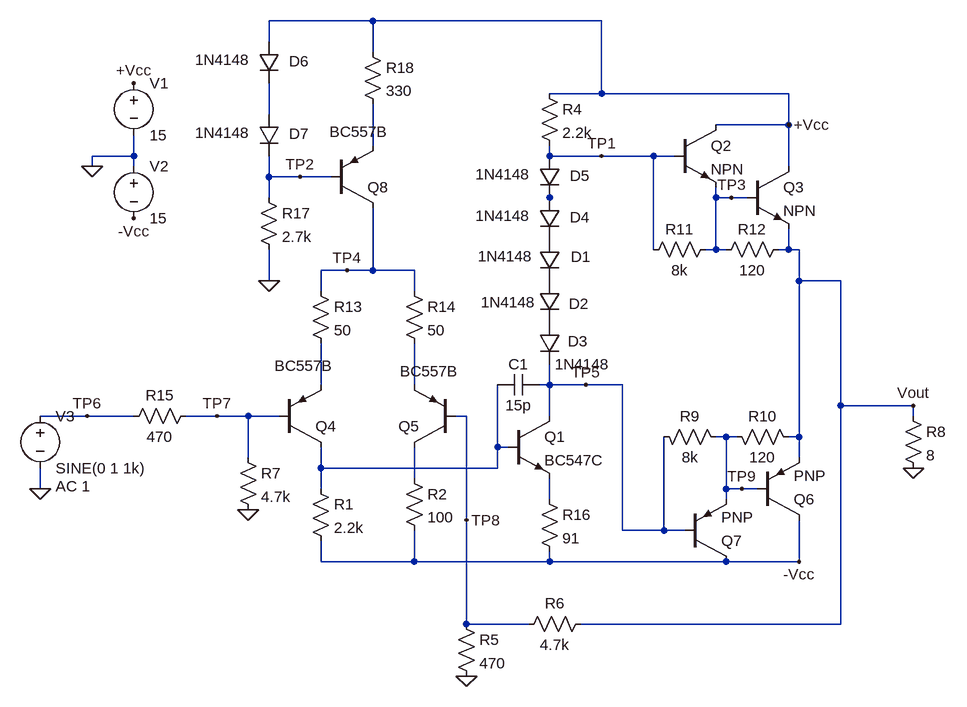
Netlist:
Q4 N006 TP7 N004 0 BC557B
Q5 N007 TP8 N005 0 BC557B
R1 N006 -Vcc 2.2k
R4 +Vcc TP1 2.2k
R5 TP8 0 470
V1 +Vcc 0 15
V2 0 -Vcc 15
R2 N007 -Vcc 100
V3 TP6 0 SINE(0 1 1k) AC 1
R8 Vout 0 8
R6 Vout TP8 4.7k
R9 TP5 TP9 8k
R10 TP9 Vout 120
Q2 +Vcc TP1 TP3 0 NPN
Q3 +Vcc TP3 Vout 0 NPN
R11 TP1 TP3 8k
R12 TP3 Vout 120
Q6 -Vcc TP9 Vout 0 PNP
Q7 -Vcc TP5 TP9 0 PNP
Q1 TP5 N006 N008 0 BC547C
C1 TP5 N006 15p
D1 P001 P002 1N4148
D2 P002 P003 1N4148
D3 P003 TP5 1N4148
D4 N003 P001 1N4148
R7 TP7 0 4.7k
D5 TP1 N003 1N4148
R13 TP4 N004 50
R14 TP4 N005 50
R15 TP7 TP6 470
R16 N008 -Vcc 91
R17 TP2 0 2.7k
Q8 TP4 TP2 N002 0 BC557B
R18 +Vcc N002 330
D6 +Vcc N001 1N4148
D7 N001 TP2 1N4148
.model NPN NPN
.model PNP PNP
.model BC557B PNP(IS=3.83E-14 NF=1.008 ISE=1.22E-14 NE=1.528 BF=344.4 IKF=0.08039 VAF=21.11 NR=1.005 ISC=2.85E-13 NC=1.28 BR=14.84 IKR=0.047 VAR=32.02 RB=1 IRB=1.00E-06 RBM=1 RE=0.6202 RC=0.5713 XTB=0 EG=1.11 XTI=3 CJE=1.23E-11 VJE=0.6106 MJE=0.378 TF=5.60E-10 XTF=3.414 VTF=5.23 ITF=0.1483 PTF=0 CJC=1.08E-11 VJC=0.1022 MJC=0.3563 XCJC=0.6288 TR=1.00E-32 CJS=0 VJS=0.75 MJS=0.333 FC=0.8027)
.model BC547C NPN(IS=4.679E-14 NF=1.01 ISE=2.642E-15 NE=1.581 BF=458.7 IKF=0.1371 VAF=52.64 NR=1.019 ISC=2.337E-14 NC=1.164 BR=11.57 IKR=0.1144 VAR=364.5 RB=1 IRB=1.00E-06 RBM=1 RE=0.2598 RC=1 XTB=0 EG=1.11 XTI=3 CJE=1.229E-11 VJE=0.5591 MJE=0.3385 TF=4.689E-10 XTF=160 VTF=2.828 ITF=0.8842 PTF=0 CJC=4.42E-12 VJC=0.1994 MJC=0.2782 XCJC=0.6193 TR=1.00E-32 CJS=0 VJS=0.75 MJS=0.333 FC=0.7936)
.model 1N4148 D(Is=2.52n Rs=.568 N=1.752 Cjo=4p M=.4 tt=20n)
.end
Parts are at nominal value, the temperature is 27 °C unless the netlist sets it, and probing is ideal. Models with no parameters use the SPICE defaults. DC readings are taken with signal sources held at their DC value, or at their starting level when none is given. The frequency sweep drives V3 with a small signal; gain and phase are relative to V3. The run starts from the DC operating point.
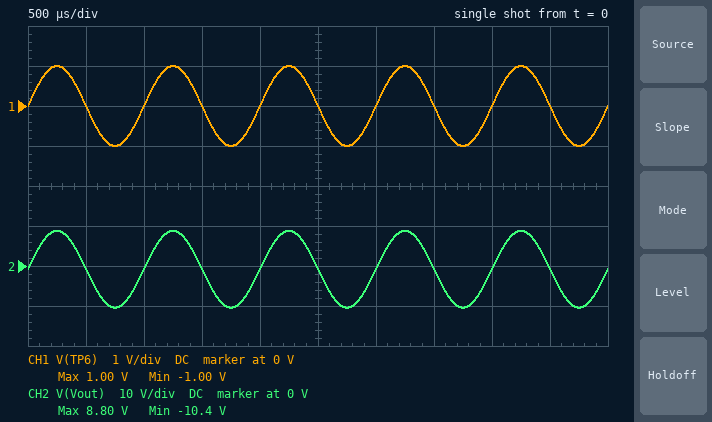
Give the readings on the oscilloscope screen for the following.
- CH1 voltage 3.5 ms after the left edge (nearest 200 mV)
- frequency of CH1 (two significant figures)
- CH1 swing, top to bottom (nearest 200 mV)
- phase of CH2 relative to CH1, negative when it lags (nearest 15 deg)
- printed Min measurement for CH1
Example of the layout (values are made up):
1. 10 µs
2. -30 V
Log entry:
1. 0 V
2. 1.0 kHz
3. 2.0 V
4. 0 deg
5. -1.00 V
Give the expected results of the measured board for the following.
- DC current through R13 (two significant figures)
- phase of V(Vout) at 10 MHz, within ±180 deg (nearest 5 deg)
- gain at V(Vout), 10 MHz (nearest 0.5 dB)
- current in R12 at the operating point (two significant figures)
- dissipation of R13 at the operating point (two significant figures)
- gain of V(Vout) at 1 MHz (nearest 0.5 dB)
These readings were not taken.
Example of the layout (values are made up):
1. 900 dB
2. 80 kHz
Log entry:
1. 580 µA
2. -110 deg
3. 13.5 dB
4. 6.7 mA
5. 17 µW
6. 19.5 dB
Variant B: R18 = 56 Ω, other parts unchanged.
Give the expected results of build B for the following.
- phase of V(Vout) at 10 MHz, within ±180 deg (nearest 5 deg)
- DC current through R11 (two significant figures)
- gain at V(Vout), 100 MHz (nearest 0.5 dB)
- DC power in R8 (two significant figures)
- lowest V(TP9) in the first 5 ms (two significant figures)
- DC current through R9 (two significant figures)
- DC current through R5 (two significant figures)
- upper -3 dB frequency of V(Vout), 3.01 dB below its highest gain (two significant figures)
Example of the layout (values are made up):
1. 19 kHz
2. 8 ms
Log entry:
1. -105 deg
2. 100 µA
3. -15.0 dB
4. 5.1 W
5. -13 V
6. 110 µA
7. 1.2 mA
8. 8.4 MHz
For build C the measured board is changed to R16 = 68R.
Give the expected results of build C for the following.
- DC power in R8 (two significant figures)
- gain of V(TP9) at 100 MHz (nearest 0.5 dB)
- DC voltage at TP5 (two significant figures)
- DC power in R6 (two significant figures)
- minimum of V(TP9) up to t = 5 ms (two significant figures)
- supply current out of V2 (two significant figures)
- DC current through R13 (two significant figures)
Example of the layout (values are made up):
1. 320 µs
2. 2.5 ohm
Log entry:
1. 100 mW
2. -17.0 dB
3. -2.6 V
4. 140 µW
5. -12 V
6. 130 mA
7. 520 µA
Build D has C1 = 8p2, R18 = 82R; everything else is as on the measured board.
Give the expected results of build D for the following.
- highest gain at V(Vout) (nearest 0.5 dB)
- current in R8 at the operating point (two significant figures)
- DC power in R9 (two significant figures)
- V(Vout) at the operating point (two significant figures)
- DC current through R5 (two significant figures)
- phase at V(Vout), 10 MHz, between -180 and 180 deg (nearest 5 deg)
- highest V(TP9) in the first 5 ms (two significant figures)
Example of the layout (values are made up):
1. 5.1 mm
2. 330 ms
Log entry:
1. 20.0 dB
2. 550 mA
3. 88 µW
4. -4.4 V
5. 840 µA
6. -80 deg
7. 4.6 V
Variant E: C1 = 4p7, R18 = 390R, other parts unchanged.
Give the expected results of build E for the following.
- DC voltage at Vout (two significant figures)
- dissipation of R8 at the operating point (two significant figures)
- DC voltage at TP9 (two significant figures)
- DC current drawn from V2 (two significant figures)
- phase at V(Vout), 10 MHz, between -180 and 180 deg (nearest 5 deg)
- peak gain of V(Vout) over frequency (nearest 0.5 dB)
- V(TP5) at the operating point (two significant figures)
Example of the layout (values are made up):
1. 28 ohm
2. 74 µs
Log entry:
1. -550 mV
2. 37 mW
3. -1.4 V
4. 88 mA
5. -70 deg
6. 20.5 dB
7. -2.3 V
